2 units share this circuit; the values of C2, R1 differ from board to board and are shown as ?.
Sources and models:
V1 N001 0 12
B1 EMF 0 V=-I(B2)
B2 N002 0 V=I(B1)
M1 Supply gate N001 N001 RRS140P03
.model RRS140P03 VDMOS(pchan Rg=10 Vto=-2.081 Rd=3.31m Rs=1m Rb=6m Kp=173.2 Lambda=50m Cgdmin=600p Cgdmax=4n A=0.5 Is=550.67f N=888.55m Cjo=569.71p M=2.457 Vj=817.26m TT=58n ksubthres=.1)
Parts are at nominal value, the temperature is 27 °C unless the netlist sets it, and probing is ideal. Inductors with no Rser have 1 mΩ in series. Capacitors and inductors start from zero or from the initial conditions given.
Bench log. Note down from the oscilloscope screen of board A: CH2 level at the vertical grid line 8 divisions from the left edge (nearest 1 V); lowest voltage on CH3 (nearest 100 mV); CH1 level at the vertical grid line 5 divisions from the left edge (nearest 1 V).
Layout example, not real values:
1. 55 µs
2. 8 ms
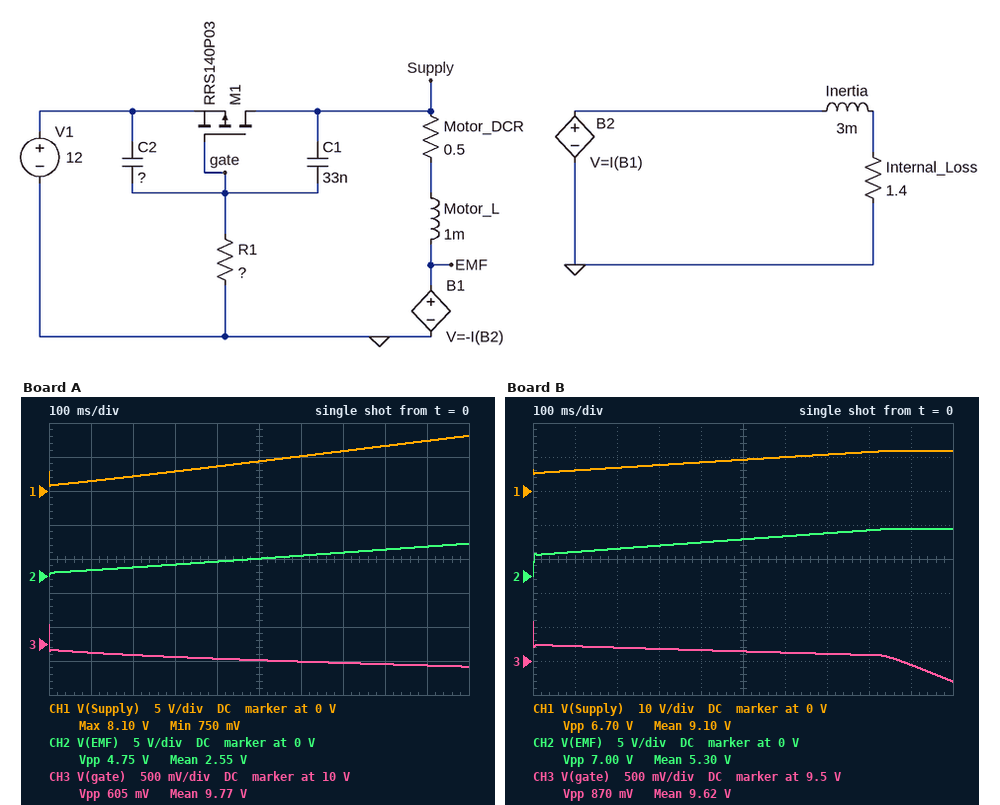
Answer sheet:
1. 4 V
2. 9.7 V
3. 4 V
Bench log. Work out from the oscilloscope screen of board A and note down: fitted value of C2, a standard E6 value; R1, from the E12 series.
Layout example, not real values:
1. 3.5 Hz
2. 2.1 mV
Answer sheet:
1. 150 nF
2. 33 MΩ
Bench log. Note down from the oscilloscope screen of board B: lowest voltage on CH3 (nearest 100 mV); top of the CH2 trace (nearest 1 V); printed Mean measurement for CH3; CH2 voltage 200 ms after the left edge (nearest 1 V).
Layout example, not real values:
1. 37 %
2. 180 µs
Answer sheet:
1. 9.2 V
2. 7 V
3. 9.62 V
4. 4 V
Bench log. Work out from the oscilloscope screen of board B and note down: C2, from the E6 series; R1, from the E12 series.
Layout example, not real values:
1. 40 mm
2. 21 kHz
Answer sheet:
1. 68 nF
2. 33 MΩ
